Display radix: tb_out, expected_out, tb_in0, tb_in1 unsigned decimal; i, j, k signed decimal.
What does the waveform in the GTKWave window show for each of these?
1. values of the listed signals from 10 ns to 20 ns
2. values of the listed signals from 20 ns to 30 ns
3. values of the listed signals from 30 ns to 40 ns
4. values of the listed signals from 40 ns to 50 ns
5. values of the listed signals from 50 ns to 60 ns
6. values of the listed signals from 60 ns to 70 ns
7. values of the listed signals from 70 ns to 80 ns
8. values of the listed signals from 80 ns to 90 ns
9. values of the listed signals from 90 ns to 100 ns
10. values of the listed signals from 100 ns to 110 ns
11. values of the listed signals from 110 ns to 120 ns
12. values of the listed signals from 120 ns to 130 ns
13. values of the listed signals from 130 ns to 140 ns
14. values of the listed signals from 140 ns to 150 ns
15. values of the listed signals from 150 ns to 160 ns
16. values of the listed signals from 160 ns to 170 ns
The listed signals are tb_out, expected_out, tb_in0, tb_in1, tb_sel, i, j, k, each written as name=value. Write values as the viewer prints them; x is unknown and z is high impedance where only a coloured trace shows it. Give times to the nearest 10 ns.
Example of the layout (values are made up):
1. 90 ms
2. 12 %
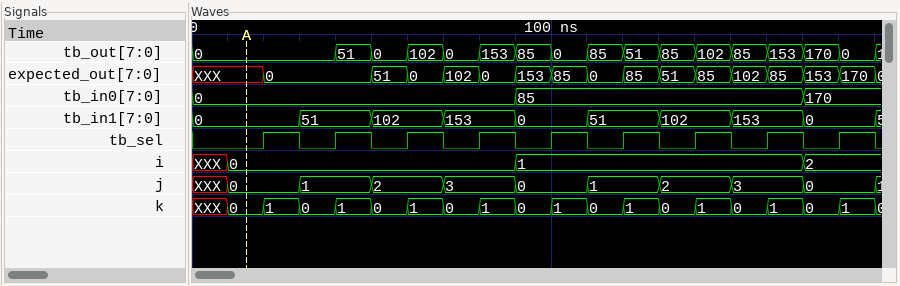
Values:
1. tb_out=0, expected_out=XXX, tb_in0=0, tb_in1=0, tb_sel=0, i=0, j=0, k=0
2. tb_out=0, expected_out=0, tb_in0=0, tb_in1=0, tb_sel=1, i=0, j=0, k=1
3. tb_out=0, expected_out=0, tb_in0=0, tb_in1=51, tb_sel=0, i=0, j=1, k=0
4. tb_out=51, expected_out=0, tb_in0=0, tb_in1=51, tb_sel=1, i=0, j=1, k=1
5. tb_out=0, expected_out=51, tb_in0=0, tb_in1=102, tb_sel=0, i=0, j=2, k=0
6. tb_out=102, expected_out=0, tb_in0=0, tb_in1=102, tb_sel=1, i=0, j=2, k=1
7. tb_out=0, expected_out=102, tb_in0=0, tb_in1=153, tb_sel=0, i=0, j=3, k=0
8. tb_out=153, expected_out=0, tb_in0=0, tb_in1=153, tb_sel=1, i=0, j=3, k=1
9. tb_out=85, expected_out=153, tb_in0=85, tb_in1=0, tb_sel=0, i=1, j=0, k=0
10. tb_out=0, expected_out=85, tb_in0=85, tb_in1=0, tb_sel=1, i=1, j=0, k=1
11. tb_out=85, expected_out=0, tb_in0=85, tb_in1=51, tb_sel=0, i=1, j=1, k=0
12. tb_out=51, expected_out=85, tb_in0=85, tb_in1=51, tb_sel=1, i=1, j=1, k=1
13. tb_out=85, expected_out=51, tb_in0=85, tb_in1=102, tb_sel=0, i=1, j=2, k=0
14. tb_out=102, expected_out=85, tb_in0=85, tb_in1=102, tb_sel=1, i=1, j=2, k=1
15. tb_out=85, expected_out=102, tb_in0=85, tb_in1=153, tb_sel=0, i=1, j=3, k=0
16. tb_out=153, expected_out=85, tb_in0=85, tb_in1=153, tb_sel=1, i=1, j=3, k=1
